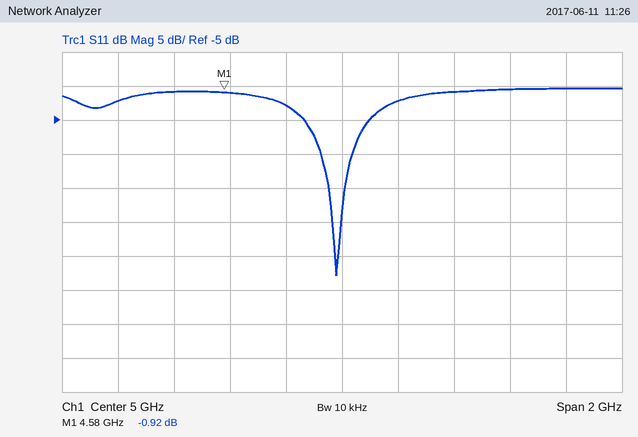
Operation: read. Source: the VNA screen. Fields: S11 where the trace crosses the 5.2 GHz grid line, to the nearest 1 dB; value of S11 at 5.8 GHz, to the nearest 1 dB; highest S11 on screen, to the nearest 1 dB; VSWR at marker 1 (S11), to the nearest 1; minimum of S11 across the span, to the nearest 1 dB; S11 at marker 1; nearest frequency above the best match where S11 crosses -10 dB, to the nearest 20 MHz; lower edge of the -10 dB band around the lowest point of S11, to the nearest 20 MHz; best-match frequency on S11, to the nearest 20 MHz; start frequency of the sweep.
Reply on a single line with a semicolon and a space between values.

-2 dB; 0 dB; 0 dB; 19; -28 dB; -0.92 dB; 5.04 GHz; 4.92 GHz; 4.98 GHz; 4 GHz
